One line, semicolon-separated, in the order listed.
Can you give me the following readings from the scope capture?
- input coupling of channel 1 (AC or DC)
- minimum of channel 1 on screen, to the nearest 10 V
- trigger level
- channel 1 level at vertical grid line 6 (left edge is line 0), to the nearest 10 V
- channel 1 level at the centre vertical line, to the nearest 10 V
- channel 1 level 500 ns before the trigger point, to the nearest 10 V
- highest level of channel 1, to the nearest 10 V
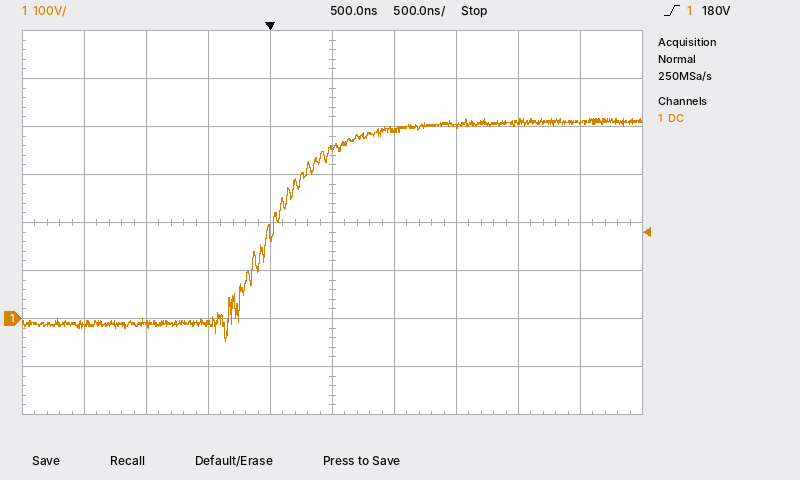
DC; -50 V; 180 V; 390 V; 350 V; -10 V; 420 V
